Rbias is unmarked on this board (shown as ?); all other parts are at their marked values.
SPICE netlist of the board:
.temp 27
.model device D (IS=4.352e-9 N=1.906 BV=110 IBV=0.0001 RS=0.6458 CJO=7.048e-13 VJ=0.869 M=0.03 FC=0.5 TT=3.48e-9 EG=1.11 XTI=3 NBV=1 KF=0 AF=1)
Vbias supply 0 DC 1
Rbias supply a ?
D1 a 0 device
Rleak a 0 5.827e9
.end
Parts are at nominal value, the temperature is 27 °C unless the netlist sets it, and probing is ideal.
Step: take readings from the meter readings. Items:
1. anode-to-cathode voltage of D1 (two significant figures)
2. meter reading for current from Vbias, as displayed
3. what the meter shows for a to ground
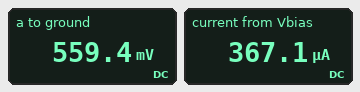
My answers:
560 mV
367.1 µA
559.4 mV
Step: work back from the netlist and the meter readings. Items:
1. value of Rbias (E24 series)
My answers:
1.2 kΩ
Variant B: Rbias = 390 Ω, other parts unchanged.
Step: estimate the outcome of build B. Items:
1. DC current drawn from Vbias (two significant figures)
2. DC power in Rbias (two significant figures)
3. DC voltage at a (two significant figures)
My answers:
1.0 mA
390 µW
610 mV
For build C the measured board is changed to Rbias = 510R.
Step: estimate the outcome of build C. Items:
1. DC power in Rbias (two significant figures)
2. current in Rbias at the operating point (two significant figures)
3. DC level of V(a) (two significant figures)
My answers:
320 µW
790 µA
600 mV
